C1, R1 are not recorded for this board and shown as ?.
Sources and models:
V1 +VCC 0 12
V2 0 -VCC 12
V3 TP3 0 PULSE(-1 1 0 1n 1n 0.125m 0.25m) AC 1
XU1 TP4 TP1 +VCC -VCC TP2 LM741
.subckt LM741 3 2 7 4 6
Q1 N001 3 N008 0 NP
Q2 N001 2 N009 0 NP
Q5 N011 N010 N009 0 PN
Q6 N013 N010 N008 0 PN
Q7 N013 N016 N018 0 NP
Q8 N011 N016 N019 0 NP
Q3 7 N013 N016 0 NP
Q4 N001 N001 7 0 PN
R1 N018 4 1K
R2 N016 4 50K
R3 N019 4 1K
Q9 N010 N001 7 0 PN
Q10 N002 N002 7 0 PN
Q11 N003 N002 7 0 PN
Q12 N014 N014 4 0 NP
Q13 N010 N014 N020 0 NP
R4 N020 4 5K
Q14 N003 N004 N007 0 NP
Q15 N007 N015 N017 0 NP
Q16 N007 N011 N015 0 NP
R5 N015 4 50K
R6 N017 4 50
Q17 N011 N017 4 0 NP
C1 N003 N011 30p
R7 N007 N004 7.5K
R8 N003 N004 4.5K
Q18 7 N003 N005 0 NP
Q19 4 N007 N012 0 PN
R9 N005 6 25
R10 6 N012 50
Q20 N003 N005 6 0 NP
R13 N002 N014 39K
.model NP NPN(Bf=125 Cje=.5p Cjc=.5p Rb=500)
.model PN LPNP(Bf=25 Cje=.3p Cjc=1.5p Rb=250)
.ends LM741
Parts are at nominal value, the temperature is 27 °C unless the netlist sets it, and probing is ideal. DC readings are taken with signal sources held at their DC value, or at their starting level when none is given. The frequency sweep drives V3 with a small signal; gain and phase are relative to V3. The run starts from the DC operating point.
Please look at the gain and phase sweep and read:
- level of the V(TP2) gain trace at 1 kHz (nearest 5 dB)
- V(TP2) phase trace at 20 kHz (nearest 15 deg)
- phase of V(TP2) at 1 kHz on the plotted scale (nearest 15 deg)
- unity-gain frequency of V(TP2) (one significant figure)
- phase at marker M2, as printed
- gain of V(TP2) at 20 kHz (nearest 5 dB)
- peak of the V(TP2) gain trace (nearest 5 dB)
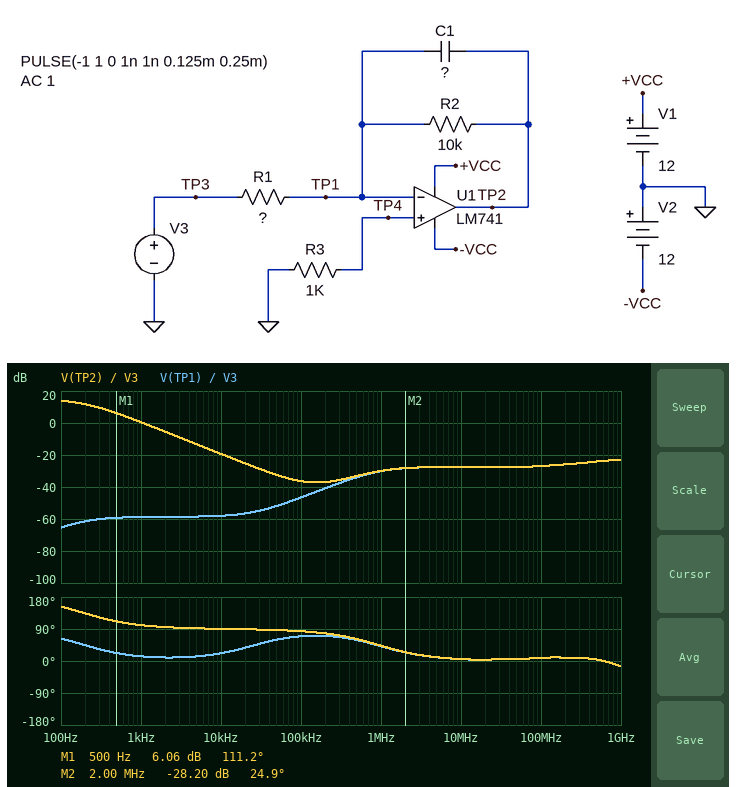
0 dB
90 deg
105 deg
1 kHz
24.9 deg
-25 dB
15 dB
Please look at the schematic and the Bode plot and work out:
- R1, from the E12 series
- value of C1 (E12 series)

1.8 kΩ
82 nF
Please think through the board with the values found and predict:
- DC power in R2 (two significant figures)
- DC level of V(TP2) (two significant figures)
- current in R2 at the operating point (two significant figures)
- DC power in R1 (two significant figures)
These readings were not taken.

3.1 mW
5.6 V
560 µA
560 µW
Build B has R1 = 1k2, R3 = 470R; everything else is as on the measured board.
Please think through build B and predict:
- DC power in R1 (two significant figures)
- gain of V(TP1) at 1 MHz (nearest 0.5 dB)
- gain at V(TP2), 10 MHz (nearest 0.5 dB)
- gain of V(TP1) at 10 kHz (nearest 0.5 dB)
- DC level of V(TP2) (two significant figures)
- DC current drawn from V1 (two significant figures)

830 µW
-28.5 dB
-26.0 dB
-54.5 dB
8.3 V
2.0 mA
